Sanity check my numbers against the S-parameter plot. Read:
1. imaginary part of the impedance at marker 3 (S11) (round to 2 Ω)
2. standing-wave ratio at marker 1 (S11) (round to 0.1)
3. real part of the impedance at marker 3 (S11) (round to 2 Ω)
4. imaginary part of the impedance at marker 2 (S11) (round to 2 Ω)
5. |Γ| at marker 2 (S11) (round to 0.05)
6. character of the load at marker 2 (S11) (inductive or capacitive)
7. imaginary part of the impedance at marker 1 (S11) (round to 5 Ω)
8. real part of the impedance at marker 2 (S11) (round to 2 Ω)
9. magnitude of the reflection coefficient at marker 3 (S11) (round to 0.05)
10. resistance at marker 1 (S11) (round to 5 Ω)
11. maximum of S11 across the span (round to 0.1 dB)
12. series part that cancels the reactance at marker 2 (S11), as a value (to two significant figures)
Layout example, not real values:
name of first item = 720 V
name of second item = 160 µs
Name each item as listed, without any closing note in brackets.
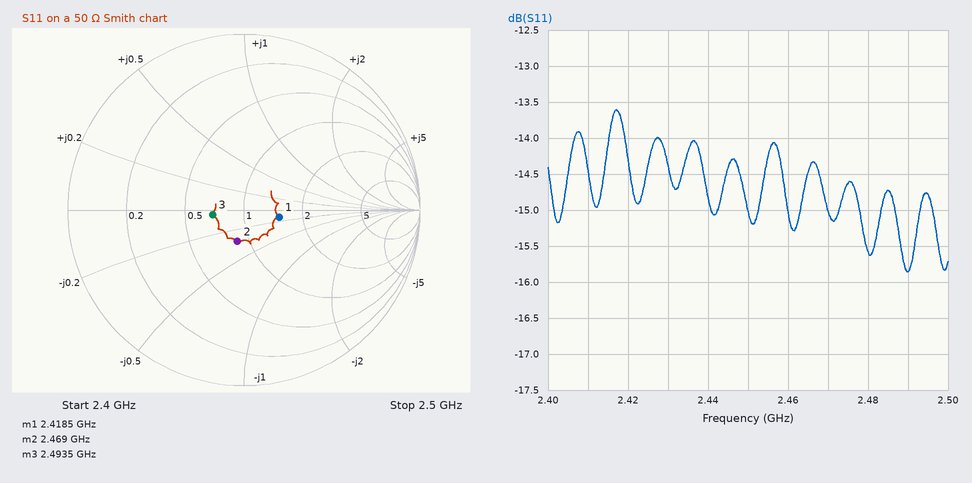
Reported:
imaginary part of the impedance at marker 3 (S11) = -2 Ω
standing-wave ratio at marker 1 (S11) = 1.5
real part of the impedance at marker 3 (S11) = 34 Ω
imaginary part of the impedance at marker 2 (S11) = -16 Ω
|Γ| at marker 2 (S11) = 0.20
character of the load at marker 2 (S11) = capacitive
imaginary part of the impedance at marker 1 (S11) = -5 Ω
real part of the impedance at marker 2 (S11) = 44 Ω
magnitude of the reflection coefficient at marker 3 (S11) = 0.20
resistance at marker 1 (S11) = 75 Ω
maximum of S11 across the span = -13.6 dB
series part that cancels the reactance at marker 2 (S11), as a value = 1.0 nH
